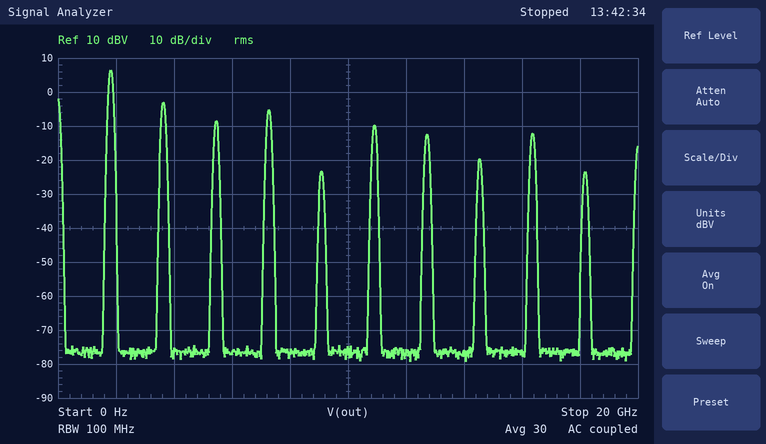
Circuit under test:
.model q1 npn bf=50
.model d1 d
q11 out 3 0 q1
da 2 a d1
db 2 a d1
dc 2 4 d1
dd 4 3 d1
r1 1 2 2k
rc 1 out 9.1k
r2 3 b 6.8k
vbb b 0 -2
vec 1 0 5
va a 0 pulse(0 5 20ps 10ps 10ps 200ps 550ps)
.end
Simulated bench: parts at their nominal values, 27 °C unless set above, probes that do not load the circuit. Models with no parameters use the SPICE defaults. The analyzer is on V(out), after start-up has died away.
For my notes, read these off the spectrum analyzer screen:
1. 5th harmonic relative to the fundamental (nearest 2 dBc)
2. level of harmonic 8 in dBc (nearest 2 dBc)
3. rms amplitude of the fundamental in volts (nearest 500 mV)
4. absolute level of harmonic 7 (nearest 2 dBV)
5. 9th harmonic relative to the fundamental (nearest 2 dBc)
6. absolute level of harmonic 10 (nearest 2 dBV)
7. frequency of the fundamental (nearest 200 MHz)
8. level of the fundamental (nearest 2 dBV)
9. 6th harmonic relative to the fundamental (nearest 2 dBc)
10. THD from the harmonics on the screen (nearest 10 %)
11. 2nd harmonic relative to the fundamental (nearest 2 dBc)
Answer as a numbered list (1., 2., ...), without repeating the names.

1. -30 dBc
2. -26 dBc
3. 2.0 V
4. -12 dBV
5. -18 dBc
6. -24 dBV
7. 1.8 GHz
8. 6 dBV
9. -16 dBc
10. 50 %
11. -10 dBc
